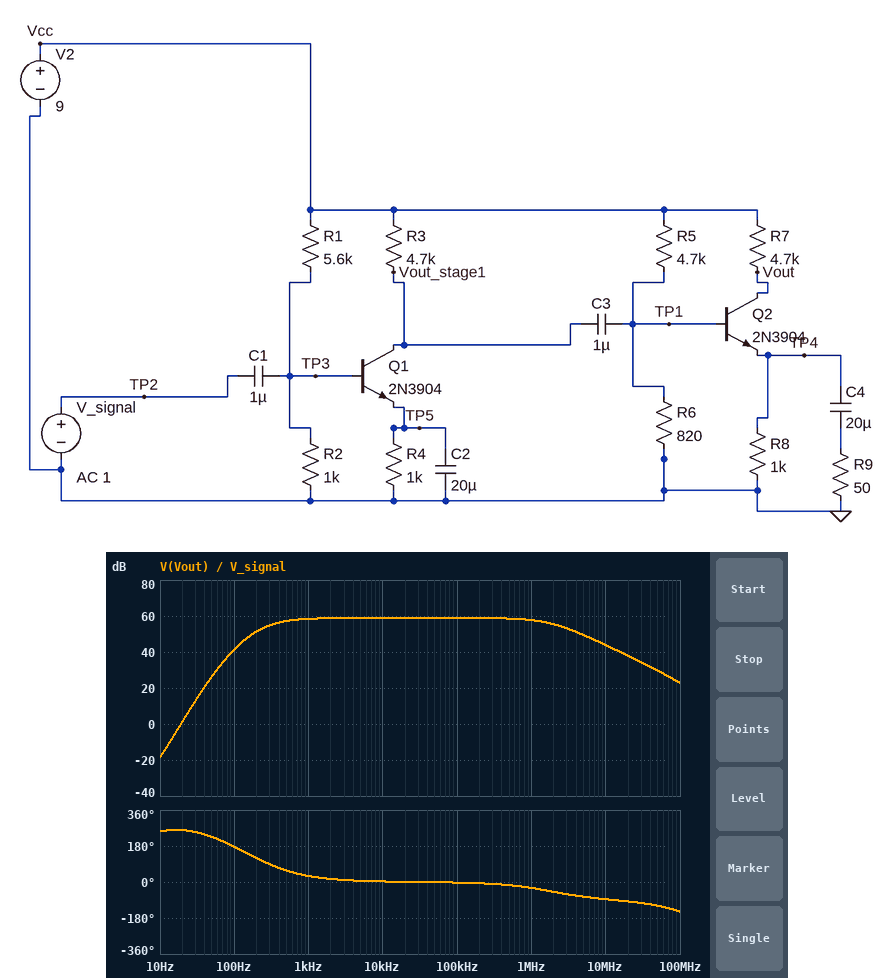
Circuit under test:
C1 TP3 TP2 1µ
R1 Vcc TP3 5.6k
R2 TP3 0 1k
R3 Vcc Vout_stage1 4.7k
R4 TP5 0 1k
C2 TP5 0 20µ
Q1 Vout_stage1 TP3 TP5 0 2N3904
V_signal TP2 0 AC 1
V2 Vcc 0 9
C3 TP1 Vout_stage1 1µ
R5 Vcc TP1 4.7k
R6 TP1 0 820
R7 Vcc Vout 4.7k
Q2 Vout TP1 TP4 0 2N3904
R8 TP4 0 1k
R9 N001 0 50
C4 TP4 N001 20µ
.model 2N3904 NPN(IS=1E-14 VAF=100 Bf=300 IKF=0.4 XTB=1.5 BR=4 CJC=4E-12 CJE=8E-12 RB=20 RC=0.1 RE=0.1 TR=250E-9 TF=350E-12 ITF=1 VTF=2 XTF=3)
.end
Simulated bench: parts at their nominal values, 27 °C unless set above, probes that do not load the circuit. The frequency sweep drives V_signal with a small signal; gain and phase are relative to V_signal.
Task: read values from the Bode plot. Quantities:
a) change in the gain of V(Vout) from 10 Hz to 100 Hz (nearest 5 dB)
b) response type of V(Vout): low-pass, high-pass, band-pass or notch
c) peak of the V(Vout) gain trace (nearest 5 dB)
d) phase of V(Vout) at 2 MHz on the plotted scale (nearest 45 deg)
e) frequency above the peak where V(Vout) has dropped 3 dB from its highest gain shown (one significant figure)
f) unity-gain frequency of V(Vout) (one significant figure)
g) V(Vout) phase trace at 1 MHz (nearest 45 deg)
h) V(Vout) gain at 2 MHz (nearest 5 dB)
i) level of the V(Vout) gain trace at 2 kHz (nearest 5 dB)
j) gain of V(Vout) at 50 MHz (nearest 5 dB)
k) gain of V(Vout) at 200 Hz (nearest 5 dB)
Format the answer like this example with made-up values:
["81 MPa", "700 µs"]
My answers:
["60 dB", "band-pass", "60 dB", "-45 deg", "2 MHz", "20 Hz", "-45 deg", "55 dB", "60 dB", "30 dB", "50 dB"]
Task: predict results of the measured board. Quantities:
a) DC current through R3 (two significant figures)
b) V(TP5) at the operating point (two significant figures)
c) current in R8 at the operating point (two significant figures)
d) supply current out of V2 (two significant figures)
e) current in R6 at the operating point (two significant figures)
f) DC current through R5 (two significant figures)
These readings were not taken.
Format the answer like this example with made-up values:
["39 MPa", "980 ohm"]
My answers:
["710 µA", "720 mV", "690 µA", "4.4 mA", "1.6 mA", "1.6 mA"]
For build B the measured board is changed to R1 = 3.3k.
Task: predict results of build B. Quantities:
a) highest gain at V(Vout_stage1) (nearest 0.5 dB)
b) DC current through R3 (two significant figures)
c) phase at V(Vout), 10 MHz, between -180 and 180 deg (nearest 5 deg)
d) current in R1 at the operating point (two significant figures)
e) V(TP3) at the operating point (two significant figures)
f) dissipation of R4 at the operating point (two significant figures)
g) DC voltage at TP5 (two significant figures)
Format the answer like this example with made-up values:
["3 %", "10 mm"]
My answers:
["30.0 dB", "1.4 mA", "-90 deg", "2.1 mA", "2.1 V", "2.0 mW", "1.4 V"]
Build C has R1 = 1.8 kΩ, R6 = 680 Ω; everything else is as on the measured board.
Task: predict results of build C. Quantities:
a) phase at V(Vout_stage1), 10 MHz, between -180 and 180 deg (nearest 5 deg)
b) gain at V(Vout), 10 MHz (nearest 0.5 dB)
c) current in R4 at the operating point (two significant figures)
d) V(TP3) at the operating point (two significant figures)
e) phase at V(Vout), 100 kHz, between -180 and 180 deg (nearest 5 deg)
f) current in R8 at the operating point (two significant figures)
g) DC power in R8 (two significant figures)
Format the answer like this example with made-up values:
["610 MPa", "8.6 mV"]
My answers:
["0 deg", "18.5 dB", "2.1 mA", "2.8 V", "-30 deg", "500 µA", "250 µW"]
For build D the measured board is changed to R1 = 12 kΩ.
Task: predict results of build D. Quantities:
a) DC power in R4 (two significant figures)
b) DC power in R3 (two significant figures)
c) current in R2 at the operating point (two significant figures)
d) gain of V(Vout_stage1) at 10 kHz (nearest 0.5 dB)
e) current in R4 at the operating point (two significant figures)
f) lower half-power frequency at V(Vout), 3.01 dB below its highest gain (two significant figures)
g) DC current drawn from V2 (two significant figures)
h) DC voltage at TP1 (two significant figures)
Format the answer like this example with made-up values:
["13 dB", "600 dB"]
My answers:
["9.8 µW", "46 µW", "690 µA", "7.0 dB", "99 µA", "220 Hz", "3.1 mA", "1.3 V"]
